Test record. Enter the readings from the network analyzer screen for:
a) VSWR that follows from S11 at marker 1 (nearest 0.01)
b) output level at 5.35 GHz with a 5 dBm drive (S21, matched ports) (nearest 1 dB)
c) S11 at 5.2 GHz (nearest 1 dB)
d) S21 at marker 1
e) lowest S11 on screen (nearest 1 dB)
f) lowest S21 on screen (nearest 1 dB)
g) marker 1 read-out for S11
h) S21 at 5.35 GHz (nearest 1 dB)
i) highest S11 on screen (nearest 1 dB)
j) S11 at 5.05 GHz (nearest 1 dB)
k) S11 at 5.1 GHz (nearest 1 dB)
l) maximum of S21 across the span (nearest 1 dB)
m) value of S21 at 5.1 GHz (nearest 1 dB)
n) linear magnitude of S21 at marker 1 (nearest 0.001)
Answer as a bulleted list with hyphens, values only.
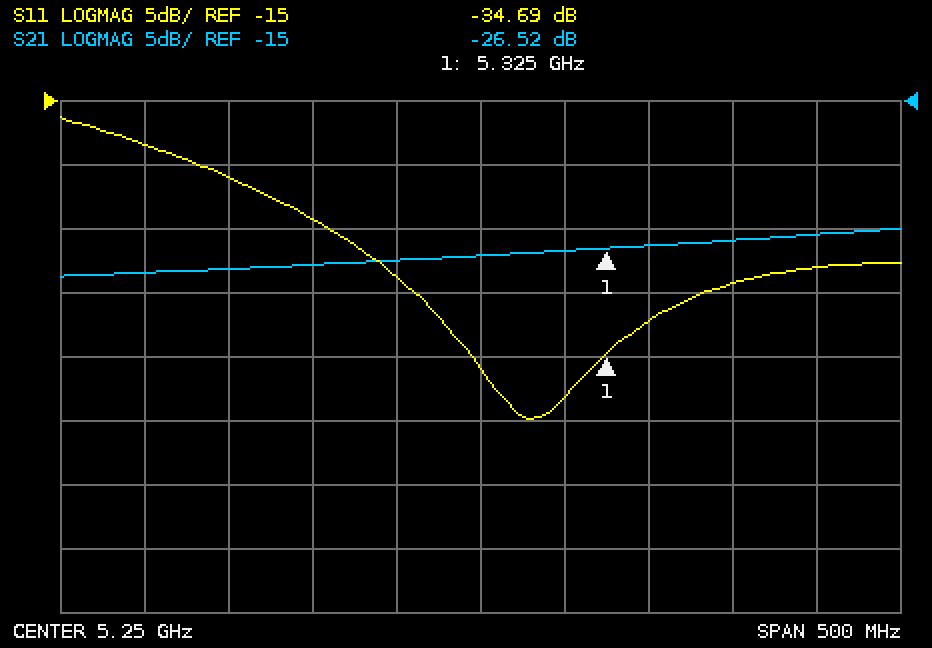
- 1.04
- -21 dBm
- -29 dB
- -26.52 dB
- -40 dB
- -29 dB
- -34.69 dB
- -26 dB
- -16 dB
- -18 dB
- -21 dB
- -25 dB
- -28 dB
- 0.047
